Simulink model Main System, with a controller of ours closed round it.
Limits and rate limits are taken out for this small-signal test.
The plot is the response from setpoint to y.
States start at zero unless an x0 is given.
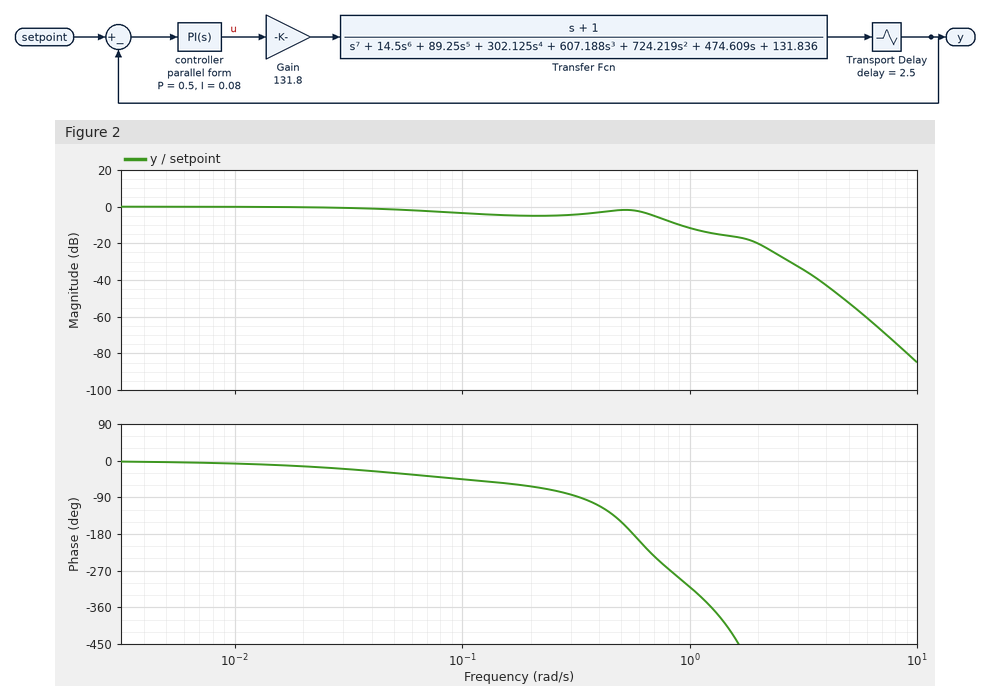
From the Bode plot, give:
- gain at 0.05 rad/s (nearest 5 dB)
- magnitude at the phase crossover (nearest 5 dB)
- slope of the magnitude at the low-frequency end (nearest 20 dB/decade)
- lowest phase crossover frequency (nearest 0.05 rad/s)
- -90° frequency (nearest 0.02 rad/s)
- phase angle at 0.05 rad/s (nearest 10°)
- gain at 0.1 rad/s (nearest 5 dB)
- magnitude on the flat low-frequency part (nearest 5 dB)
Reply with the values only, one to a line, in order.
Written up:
0 dB
0 dB
0 dB/decade
0.55 rad/s
0.32 rad/s
-30°
-5 dB
0 dB
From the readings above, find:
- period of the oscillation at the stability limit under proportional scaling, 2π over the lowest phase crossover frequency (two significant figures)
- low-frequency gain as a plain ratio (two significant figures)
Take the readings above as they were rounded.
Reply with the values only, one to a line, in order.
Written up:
11 s
1.0
